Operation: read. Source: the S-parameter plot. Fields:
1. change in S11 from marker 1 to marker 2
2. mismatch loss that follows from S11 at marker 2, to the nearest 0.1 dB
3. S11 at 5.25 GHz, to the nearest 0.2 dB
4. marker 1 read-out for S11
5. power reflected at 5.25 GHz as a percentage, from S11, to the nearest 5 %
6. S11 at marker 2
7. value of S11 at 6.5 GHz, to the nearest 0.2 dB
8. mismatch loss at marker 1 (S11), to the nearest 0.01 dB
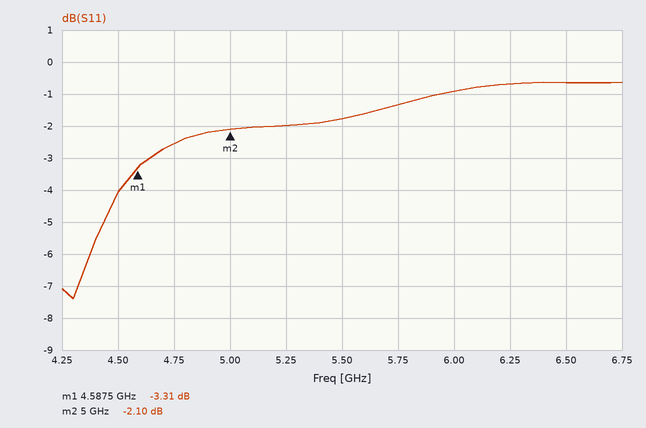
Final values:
1.21 dB
4.2 dB
-2.0 dB
-3.31 dB
65 %
-2.10 dB
-0.6 dB
2.73 dB
